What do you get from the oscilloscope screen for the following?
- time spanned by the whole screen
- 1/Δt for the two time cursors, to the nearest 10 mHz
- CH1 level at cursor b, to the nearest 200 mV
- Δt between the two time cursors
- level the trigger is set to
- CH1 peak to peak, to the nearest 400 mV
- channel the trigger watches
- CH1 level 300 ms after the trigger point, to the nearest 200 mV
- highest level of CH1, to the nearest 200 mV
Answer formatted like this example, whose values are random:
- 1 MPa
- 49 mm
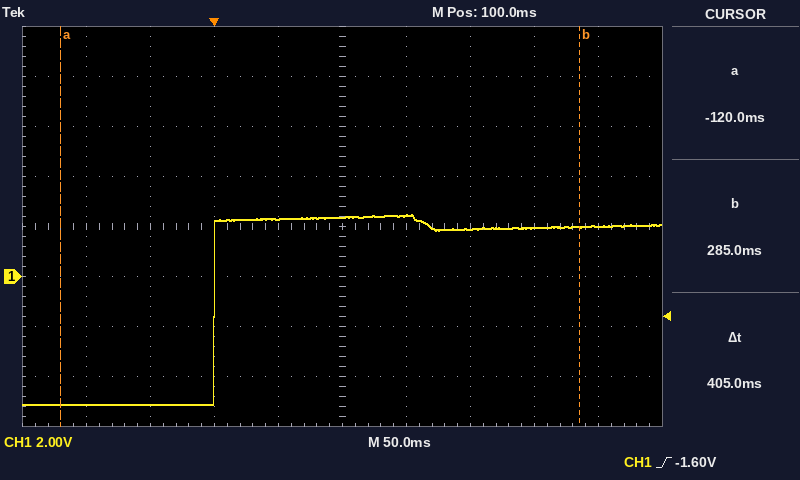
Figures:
- 500 ms
- 2.47 Hz
- 2.0 V
- 405 ms
- -1.60 V
- 7.6 V
- CH1
- 2.0 V
- 2.4 V
